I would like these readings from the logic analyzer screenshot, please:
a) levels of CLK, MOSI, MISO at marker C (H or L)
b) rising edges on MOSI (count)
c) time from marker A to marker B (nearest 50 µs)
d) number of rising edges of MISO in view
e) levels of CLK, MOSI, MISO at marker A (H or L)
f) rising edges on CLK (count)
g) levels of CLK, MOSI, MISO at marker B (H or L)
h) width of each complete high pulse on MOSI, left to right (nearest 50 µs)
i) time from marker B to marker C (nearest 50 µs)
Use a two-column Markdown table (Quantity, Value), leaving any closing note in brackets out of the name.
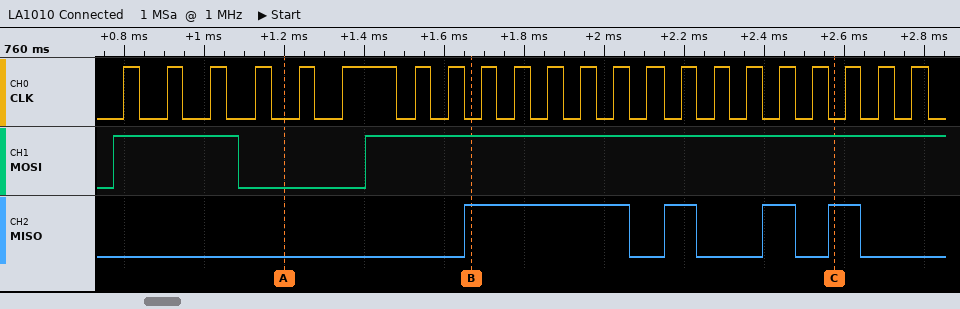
| Quantity | Value |
|---|---|
| levels of CLK, MOSI, MISO at marker C | CLK=L, MOSI=H, MISO=H |
| rising edges on MOSI | 2 |
| time from marker A to marker B | 450 µs |
| number of rising edges of MISO in view | 4 |
| levels of CLK, MOSI, MISO at marker A | CLK=L, MOSI=L, MISO=L |
| rising edges on CLK | 22 |
| levels of CLK, MOSI, MISO at marker B | CLK=L, MOSI=H, MISO=H |
| width of each complete high pulse on MOSI, left to right | 300 µs |
| time from marker B to marker C | 900 µs |
